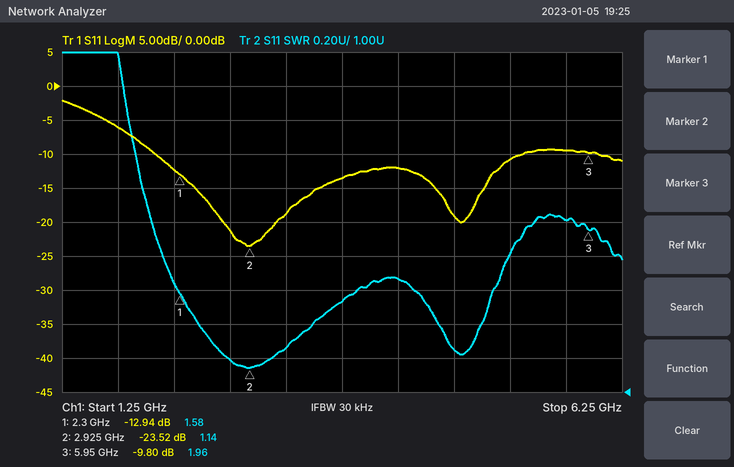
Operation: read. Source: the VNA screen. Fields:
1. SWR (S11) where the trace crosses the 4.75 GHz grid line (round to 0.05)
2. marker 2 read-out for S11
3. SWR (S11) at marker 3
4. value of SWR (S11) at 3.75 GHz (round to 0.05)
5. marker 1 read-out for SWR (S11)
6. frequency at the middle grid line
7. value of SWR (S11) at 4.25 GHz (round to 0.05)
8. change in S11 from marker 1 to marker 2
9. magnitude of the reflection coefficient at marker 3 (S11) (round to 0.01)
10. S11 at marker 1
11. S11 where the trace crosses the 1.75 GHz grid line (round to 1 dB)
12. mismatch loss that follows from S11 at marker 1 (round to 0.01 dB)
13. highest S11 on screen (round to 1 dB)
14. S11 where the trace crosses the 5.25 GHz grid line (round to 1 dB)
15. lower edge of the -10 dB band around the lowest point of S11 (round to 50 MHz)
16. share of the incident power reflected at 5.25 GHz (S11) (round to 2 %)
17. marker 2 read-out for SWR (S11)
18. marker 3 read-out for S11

1.25
-23.52 dB
1.96
1.55
1.58
3.75 GHz
1.65
-10.58 dB
0.32
-12.94 dB
-6 dB
0.23 dB
-2 dB
-11 dB
2.10 GHz
8 %
1.14
-9.80 dB
